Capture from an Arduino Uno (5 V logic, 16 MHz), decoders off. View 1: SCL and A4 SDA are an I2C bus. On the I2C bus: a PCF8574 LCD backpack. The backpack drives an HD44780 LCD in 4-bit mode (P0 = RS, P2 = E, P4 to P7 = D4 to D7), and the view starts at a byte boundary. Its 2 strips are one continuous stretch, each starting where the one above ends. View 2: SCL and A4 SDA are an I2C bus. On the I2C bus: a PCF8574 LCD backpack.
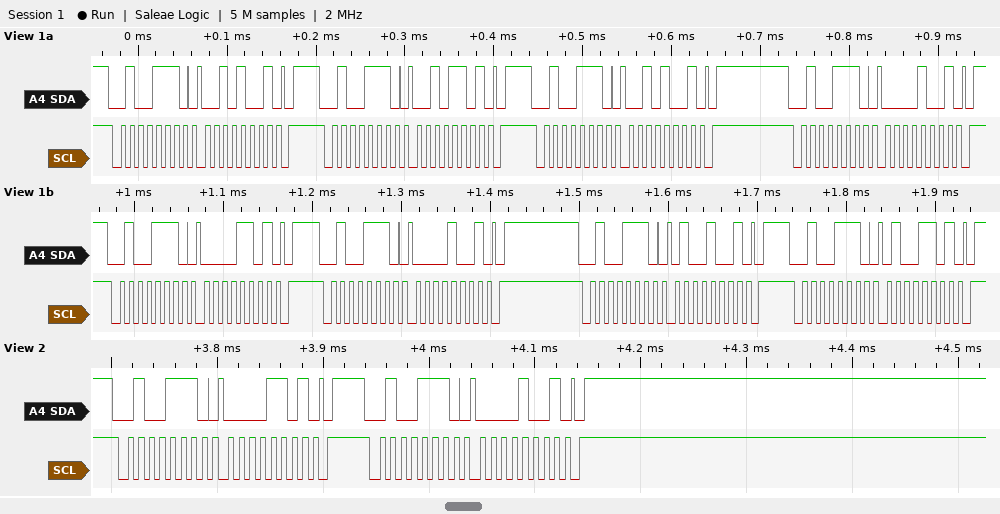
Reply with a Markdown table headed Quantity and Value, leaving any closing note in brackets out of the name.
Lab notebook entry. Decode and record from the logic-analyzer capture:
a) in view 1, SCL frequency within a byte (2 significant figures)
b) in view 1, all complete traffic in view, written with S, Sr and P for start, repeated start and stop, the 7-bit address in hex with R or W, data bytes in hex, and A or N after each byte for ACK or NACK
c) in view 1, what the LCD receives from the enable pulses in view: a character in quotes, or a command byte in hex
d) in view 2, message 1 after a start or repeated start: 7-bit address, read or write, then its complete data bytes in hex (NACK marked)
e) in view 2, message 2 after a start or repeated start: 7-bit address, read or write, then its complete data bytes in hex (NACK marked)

| Quantity | Value |
|---|---|
| in view 1, SCL frequency within a byte | 100 kHz |
| in view 1, all complete traffic in view, written with S, Sr and P for start, repeated start and stop, the 7-bit address in hex with R or W, data bytes in hex, and A or N after each byte for ACK or NACK | S 27W A 29 A P S 27W A 2D A P S 27W A 29 A P S 27W A 09 A P S 27W A 0D A P S 27W A 09 A P S 27W A 49 A P S 27W A 4D A P |
| in view 1, what the LCD receives from the enable pulses in view: a character in quotes, or a command byte in hex | ' ' |
| in view 2, message 1 after a start or repeated start: 7-bit address, read or write, then its complete data bytes in hex | 0x27 write: 0D |
| in view 2, message 2 after a start or repeated start: 7-bit address, read or write, then its complete data bytes in hex | 0x27 write: 09 |
